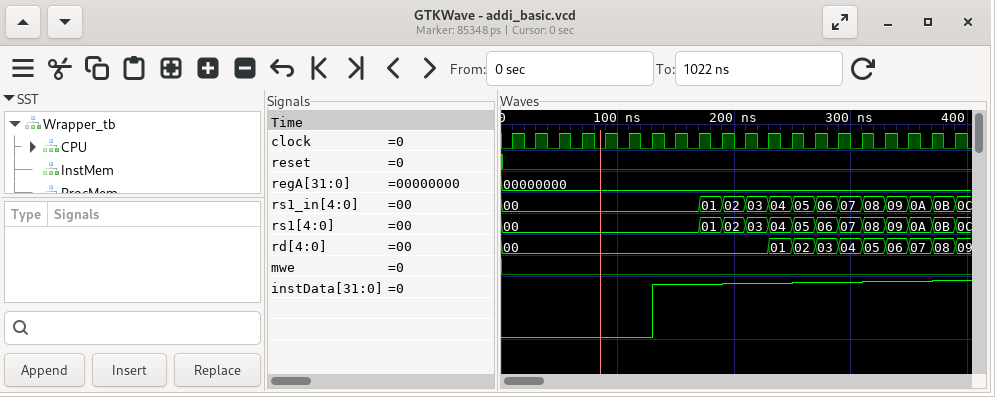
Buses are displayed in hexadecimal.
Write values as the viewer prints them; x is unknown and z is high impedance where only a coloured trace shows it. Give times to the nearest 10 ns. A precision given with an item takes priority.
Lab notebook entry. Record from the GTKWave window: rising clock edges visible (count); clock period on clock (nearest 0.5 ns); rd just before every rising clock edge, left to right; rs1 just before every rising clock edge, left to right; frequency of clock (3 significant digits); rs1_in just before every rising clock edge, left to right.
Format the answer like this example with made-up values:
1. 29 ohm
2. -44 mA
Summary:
1. 20
2. 20 ns
3. 00, 00, 00, 00, 00, 00, 00, 00, 00, 00, 00, 00, 01, 02, 03, 04, 05, 06, 07, 08
4. 00, 00, 00, 00, 00, 00, 00, 00, 00, 01, 02, 03, 04, 05, 06, 07, 08, 09, 0A, 0B
5. 50.0 MHz
6. 00, 00, 00, 00, 00, 00, 00, 00, 00, 01, 02, 03, 04, 05, 06, 07, 08, 09, 0A, 0B
